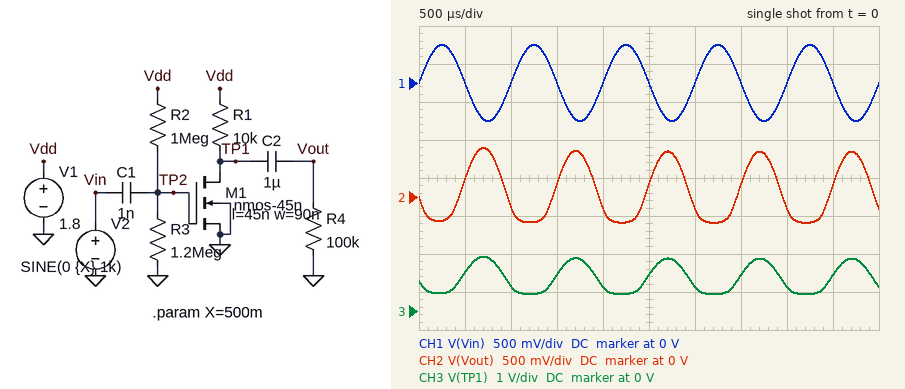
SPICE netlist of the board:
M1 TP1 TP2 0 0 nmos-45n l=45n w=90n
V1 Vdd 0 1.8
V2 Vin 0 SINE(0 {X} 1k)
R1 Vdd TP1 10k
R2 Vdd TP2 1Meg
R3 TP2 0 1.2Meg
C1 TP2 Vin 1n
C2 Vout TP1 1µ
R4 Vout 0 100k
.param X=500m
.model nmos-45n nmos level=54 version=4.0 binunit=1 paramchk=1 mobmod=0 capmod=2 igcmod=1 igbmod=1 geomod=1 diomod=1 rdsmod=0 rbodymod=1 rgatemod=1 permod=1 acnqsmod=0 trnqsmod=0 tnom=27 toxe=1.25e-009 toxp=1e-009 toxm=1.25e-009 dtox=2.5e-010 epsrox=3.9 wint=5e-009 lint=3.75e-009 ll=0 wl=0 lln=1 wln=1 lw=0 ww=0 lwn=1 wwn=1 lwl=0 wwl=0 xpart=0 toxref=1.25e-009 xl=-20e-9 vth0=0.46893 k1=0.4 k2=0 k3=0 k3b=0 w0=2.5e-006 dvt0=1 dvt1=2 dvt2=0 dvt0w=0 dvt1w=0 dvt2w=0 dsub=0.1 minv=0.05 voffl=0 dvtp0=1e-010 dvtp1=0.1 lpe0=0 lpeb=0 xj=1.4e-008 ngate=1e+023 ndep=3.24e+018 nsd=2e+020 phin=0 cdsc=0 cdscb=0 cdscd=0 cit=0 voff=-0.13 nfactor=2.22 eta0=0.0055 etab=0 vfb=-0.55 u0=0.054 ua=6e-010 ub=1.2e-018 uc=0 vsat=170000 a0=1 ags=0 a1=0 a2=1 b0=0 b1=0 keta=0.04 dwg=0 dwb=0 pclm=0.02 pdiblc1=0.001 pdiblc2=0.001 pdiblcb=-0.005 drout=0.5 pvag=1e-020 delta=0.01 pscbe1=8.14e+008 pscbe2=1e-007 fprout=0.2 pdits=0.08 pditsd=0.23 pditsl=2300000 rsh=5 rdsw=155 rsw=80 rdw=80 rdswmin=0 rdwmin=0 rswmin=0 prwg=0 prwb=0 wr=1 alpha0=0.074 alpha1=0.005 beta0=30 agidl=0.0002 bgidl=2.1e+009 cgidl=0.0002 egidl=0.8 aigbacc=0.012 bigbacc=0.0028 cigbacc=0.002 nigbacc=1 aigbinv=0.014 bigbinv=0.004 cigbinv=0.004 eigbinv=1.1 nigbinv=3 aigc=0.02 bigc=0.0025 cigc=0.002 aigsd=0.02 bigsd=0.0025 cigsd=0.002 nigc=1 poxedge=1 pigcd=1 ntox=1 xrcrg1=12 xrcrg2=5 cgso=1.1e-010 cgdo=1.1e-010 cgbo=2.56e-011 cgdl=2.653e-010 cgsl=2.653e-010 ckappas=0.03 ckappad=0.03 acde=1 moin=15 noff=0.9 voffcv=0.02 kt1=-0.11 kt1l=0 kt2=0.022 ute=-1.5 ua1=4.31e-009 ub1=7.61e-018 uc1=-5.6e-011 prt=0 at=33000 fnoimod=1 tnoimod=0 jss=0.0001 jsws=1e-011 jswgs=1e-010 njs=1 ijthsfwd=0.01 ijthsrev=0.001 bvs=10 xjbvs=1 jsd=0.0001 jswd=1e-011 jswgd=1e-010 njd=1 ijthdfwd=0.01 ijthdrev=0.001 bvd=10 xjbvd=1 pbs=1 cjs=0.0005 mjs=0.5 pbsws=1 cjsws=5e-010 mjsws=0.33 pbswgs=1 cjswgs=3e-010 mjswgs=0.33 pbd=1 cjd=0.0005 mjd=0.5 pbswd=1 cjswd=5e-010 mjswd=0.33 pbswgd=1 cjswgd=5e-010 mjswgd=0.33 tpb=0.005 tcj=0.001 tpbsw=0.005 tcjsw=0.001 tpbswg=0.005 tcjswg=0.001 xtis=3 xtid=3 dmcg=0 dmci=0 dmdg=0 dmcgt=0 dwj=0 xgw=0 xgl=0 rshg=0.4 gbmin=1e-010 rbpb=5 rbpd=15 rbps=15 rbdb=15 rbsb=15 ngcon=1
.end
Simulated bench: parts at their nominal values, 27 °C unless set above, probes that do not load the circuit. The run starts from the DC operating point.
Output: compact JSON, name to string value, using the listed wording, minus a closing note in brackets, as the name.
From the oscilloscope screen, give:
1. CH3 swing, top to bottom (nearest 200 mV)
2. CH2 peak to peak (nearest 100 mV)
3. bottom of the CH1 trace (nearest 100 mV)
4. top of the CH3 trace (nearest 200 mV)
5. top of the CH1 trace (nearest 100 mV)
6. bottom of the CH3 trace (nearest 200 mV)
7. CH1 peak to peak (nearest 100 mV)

{"CH3 swing, top to bottom": "1.0 V", "CH2 peak to peak": "1.0 V", "bottom of the CH1 trace": "-500 mV", "top of the CH3 trace": "1.4 V", "top of the CH1 trace": "500 mV", "bottom of the CH3 trace": "400 mV", "CH1 peak to peak": "1.0 V"}
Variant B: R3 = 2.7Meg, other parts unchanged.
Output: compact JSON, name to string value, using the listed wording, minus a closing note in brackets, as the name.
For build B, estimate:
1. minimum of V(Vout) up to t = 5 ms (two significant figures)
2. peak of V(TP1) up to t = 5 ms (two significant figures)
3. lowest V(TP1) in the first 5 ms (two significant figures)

{"minimum of V(Vout) up to t = 5 ms": "-79 mV", "peak of V(TP1) up to t = 5 ms": "1.0 V", "lowest V(TP1) in the first 5 ms": "400 mV"}
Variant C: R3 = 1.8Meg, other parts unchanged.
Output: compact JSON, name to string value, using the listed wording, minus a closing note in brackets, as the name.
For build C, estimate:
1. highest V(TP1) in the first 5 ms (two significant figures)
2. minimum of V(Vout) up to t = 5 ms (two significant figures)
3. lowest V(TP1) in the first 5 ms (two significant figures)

{"highest V(TP1) in the first 5 ms": "1.2 V", "minimum of V(Vout) up to t = 5 ms": "-170 mV", "lowest V(TP1) in the first 5 ms": "410 mV"}
